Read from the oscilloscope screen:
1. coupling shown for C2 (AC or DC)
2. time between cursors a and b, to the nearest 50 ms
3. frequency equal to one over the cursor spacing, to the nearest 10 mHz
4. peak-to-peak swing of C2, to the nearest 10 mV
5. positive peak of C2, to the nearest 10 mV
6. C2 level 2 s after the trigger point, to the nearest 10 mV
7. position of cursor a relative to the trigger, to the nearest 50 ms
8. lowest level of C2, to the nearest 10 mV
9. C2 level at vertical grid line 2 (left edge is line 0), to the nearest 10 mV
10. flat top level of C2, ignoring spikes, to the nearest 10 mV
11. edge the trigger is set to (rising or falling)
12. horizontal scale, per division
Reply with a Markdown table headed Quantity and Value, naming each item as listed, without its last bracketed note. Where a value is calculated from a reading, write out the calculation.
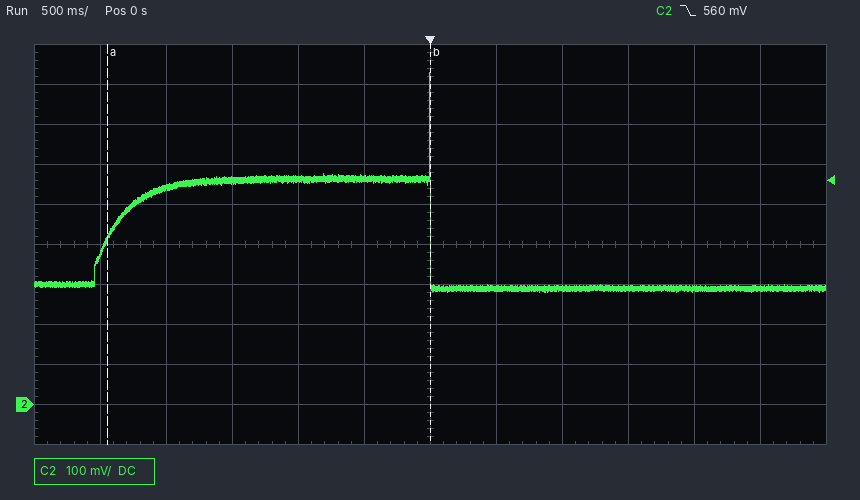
| Quantity | Value |
|---|---|
| coupling shown for C2 | DC |
| time between cursors a and b, to the nearest 50 ms | 2.45 s |
| frequency equal to one over the cursor spacing, to the nearest 10 mHz | 1 / 2.45 s ≈ 410 mHz |
| peak-to-peak swing of C2, to the nearest 10 mV | 830 mV − (280 mV) = 550 mV |
| positive peak of C2, to the nearest 10 mV | 830 mV |
| C2 level 2 s after the trigger point, to the nearest 10 mV | 290 mV |
| position of cursor a relative to the trigger, to the nearest 50 ms | -2.45 s |
| lowest level of C2, to the nearest 10 mV | 280 mV |
| C2 level at vertical grid line 2 (left edge is line 0), to the nearest 10 mV | 540 mV |
| flat top level of C2, ignoring spikes, to the nearest 10 mV | 560 mV |
| edge the trigger is set to | falling |
| horizontal scale, per division | 500 ms |
